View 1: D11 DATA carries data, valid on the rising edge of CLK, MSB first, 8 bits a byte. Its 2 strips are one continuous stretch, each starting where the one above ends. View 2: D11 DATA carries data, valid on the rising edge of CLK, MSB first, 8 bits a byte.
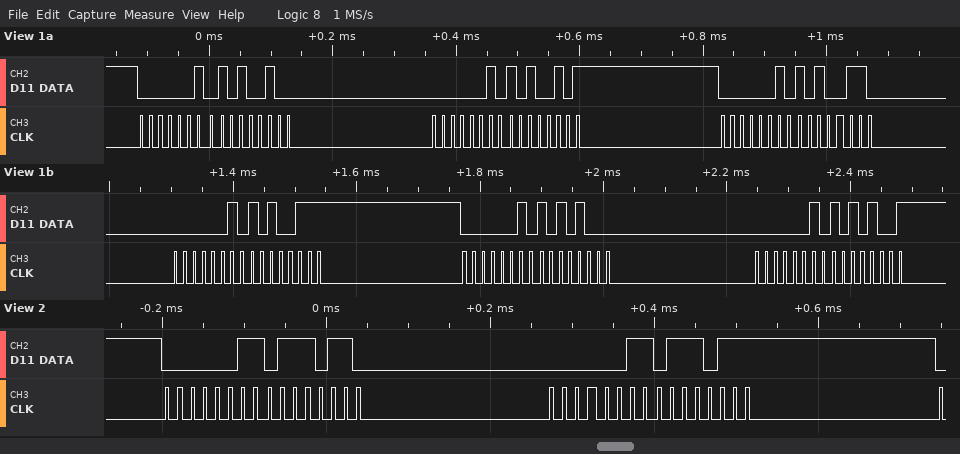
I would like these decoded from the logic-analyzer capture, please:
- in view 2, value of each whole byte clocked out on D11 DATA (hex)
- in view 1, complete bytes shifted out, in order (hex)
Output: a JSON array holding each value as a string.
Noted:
["0x03 0x76 0x03 0x77", "02 A4 02 A5 02 A6 02 A7 02 A8 02 A9"]
